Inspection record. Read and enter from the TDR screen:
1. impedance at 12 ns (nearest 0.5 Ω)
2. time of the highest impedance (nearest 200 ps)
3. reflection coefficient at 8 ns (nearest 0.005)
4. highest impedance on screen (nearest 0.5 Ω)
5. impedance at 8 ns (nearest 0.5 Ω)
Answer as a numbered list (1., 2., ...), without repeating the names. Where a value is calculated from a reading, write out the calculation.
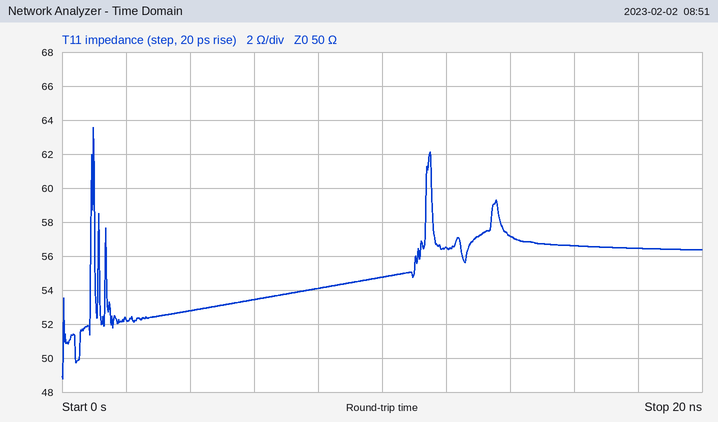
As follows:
1. 56.5 Ω
2. 1.0 ns
3. (54 − 50)/(54 + 50) ≈ +0.0385, so +0.040 to the nearest 0.005
4. 63.5 Ω
5. 54.0 Ω
